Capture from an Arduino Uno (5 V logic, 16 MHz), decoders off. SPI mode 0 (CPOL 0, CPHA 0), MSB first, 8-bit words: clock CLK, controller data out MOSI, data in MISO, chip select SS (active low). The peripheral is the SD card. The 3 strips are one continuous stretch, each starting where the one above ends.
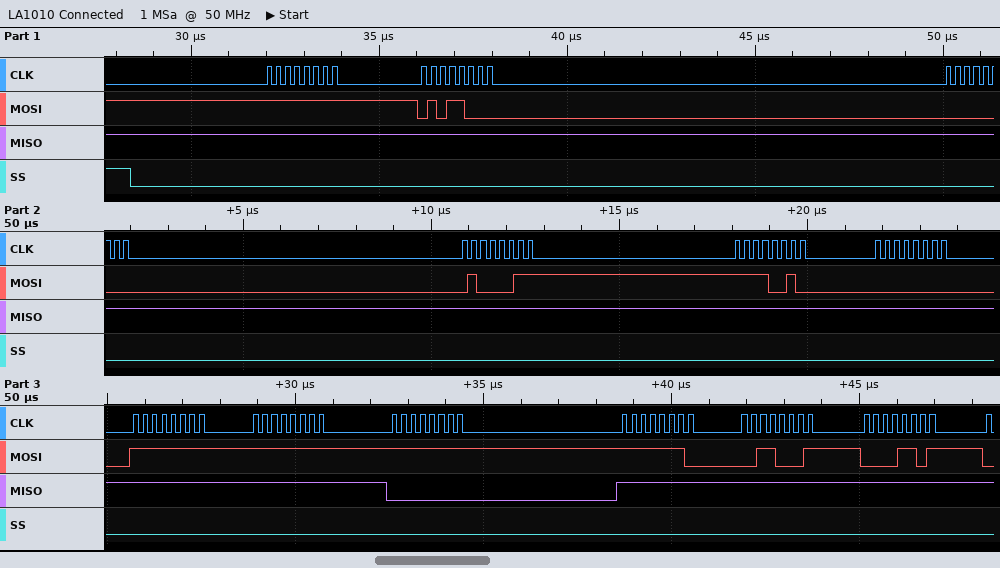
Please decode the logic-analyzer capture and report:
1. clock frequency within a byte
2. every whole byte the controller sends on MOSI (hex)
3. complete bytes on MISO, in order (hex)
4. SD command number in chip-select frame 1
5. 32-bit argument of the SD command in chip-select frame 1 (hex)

4 MHz
FF 58 00 43 F2 00 FF FF FF FE 31 0D
FF FF FF FF FF FF FF FF 00 FF FF FF
CMD24
0x0043F200
